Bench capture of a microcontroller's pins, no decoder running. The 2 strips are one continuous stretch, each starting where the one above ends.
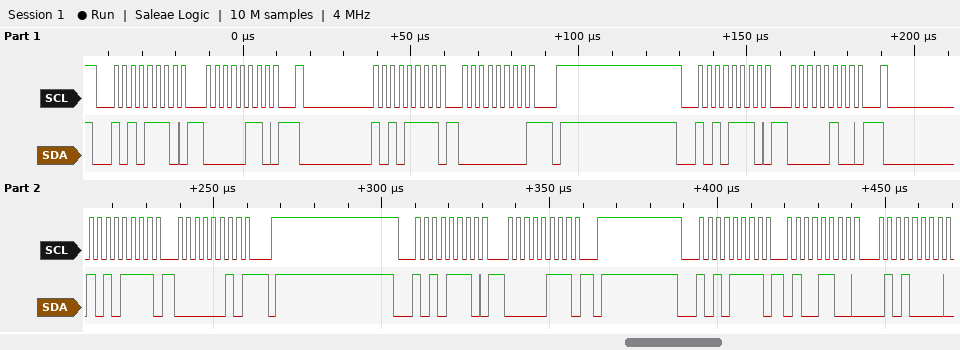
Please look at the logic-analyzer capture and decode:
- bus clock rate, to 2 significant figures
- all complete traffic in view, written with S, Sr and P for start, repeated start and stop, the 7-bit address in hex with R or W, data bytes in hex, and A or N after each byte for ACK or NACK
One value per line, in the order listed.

400 kHz
S 57W A 06 A Sr 57R A 00 N P S 57W A 04 A Sr 57R A 02 N P S 57W A 07 A P S 57R A 4C A 50 A
